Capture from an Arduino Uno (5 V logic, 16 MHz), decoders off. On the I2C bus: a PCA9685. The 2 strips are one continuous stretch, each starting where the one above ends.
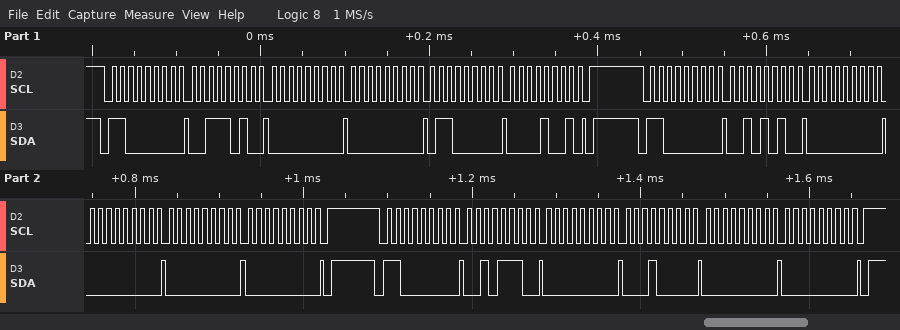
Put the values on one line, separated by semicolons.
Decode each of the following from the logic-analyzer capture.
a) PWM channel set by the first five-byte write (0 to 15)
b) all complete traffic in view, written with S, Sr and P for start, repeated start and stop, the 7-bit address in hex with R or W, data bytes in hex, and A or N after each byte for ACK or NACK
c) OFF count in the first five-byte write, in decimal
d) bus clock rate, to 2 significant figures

13; S 60W A 3A A 00 A 00 A 60 A 09 A P S 60W A 2A A 00 A 00 A 00 A 00 A P S 60W A 2E A 00 A 10 A 00 A 00 A P; 2400; 100 kHz
